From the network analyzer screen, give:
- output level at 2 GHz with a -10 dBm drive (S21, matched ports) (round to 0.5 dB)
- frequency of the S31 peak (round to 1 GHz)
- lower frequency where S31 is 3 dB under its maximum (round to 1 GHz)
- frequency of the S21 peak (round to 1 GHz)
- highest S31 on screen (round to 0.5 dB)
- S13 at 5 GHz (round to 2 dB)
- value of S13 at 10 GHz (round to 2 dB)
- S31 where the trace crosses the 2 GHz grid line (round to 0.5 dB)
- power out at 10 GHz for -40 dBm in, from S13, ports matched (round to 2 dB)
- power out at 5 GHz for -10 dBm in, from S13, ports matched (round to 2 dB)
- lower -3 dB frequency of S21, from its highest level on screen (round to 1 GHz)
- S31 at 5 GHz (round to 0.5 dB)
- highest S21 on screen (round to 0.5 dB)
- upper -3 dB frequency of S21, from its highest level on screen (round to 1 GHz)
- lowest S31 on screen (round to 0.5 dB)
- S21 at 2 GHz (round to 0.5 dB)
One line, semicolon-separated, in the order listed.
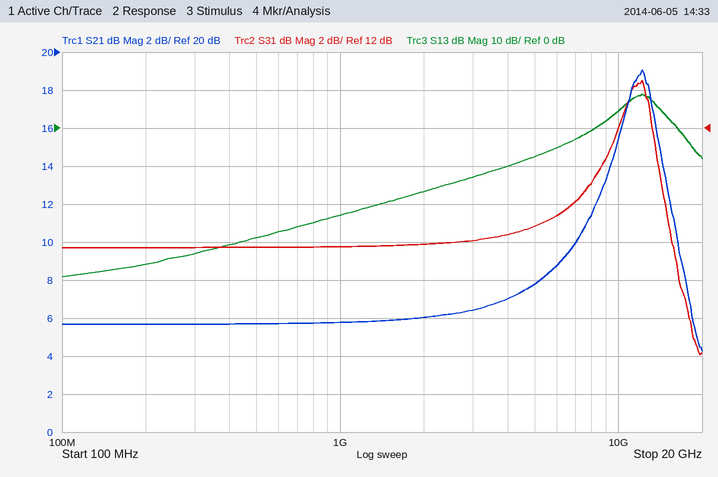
-4.0 dBm; 12 GHz; 10 GHz; 12 GHz; 14.5 dB; -8 dB; 4 dB; 6.0 dB; -36 dBm; -18 dBm; 10 GHz; 7.0 dB; 19.0 dB; 14 GHz; 0.0 dB; 6.0 dB
